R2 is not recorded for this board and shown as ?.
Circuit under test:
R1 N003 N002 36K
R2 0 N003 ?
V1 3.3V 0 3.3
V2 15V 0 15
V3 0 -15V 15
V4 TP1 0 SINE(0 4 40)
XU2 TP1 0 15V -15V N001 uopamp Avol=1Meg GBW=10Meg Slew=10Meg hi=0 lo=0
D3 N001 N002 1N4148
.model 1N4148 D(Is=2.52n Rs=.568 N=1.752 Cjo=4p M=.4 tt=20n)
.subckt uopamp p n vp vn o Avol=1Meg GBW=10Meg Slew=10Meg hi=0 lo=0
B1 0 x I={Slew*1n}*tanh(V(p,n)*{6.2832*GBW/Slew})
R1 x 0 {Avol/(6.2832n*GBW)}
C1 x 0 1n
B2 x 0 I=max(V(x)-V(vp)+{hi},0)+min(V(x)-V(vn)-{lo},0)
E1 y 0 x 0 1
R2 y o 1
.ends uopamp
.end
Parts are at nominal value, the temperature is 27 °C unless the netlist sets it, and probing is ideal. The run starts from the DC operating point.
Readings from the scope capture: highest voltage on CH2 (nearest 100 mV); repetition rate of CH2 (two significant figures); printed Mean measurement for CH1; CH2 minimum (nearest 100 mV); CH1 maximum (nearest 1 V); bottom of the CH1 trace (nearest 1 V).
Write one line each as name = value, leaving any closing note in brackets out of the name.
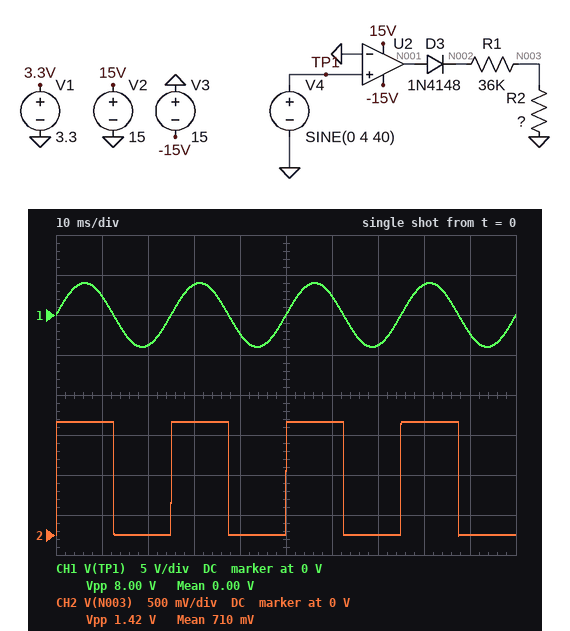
highest voltage on CH2 = 1.4 V
repetition rate of CH2 = 40 Hz
printed Mean measurement for CH1 = 0.00 V
CH2 minimum = 0 V
CH1 maximum = 4 V
bottom of the CH1 trace = -4 V
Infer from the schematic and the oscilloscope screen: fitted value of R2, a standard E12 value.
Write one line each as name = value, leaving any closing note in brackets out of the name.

fitted value of R2, a standard E12 value = 3.9 kΩ
